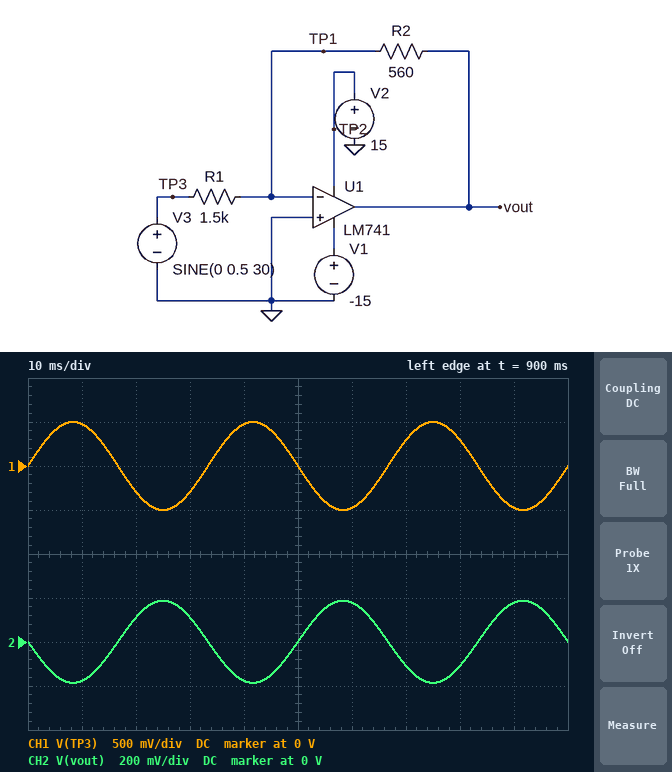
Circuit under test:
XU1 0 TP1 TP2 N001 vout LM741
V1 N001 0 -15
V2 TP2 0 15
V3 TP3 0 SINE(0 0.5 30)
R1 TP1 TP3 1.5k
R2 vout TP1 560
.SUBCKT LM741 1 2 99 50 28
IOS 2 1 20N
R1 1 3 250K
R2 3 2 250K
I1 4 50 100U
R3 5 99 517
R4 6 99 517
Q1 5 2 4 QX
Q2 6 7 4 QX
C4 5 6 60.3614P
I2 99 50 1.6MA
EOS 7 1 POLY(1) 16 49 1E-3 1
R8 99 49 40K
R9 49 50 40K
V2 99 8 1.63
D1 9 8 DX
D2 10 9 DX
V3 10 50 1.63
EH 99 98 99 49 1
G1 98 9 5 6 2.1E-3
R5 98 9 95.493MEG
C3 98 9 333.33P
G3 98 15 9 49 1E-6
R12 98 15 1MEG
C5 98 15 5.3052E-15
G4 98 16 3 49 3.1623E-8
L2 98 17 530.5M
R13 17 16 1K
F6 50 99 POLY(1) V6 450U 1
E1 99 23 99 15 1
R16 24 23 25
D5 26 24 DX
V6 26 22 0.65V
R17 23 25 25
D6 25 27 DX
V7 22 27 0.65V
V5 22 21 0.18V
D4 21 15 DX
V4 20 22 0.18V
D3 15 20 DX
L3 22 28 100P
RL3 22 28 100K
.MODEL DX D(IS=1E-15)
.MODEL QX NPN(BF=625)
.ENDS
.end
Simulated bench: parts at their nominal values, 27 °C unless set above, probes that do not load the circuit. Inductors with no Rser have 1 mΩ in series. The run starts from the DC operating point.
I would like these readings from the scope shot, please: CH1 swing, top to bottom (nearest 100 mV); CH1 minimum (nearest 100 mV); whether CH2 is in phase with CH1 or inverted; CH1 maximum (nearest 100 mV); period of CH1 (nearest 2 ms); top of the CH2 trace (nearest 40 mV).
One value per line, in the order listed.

1.0 V
-500 mV
inverted
500 mV
34 ms
200 mV
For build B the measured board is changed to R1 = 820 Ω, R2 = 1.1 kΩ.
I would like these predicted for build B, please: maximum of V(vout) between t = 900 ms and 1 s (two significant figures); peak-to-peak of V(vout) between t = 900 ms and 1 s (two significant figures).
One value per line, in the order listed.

670 mV
1.3 V
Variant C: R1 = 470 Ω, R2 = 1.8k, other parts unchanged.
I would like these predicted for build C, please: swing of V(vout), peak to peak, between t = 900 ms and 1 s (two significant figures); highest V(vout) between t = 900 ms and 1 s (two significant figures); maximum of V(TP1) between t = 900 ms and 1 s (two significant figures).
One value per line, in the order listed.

3.8 V
1.9 V
1.1 mV
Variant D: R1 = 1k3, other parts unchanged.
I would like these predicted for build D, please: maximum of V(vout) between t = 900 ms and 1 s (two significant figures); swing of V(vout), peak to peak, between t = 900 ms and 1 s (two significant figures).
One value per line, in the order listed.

220 mV
430 mV
